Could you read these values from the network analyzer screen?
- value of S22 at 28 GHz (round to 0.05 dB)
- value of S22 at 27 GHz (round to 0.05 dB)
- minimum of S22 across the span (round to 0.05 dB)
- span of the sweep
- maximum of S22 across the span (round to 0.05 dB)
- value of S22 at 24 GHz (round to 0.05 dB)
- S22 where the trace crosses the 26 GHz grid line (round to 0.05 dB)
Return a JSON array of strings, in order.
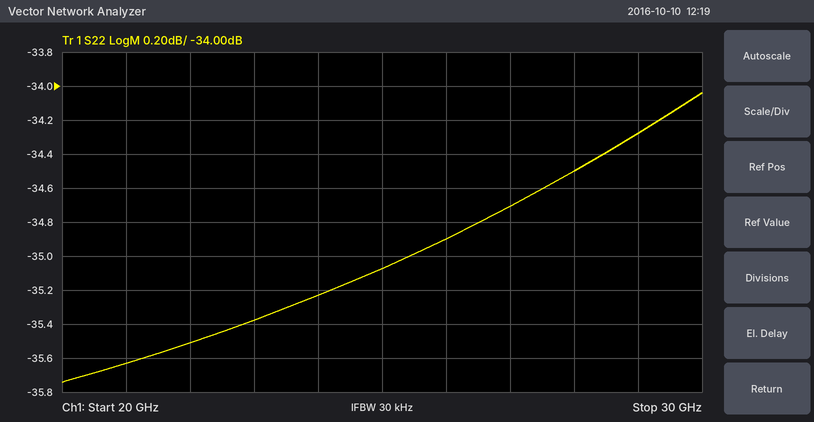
["-34.50 dB", "-34.70 dB", "-35.75 dB", "10 GHz", "-34.05 dB", "-35.25 dB", "-34.90 dB"]
